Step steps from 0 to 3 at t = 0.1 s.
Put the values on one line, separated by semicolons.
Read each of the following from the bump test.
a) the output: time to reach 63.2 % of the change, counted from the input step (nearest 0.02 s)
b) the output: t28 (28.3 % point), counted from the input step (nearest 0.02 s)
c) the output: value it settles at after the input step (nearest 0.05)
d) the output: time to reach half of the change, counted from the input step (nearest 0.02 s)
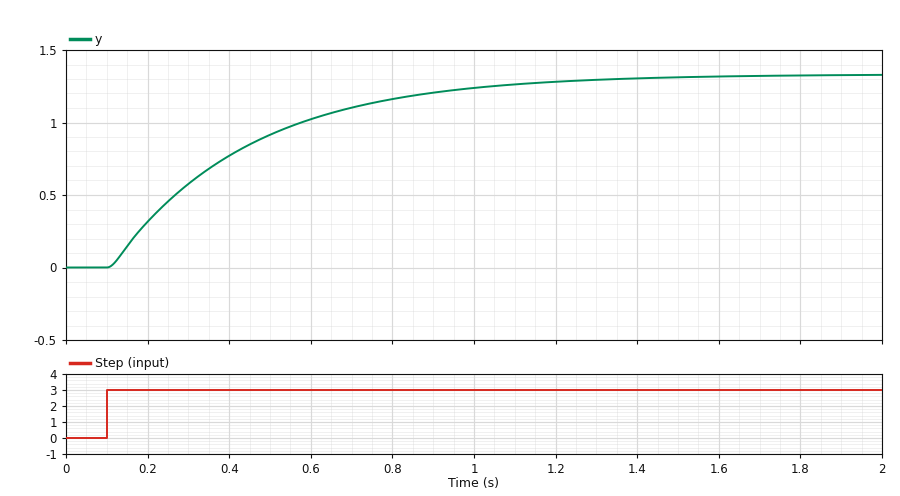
0.34 s; 0.12 s; 1.35; 0.24 s
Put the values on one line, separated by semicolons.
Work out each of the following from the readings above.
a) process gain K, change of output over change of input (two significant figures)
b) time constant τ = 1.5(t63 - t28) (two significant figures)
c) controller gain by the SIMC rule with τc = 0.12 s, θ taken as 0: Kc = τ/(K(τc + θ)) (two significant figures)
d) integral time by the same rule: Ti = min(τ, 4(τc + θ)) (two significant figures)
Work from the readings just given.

0.45; 0.33 s; 6.1; 0.33 s
